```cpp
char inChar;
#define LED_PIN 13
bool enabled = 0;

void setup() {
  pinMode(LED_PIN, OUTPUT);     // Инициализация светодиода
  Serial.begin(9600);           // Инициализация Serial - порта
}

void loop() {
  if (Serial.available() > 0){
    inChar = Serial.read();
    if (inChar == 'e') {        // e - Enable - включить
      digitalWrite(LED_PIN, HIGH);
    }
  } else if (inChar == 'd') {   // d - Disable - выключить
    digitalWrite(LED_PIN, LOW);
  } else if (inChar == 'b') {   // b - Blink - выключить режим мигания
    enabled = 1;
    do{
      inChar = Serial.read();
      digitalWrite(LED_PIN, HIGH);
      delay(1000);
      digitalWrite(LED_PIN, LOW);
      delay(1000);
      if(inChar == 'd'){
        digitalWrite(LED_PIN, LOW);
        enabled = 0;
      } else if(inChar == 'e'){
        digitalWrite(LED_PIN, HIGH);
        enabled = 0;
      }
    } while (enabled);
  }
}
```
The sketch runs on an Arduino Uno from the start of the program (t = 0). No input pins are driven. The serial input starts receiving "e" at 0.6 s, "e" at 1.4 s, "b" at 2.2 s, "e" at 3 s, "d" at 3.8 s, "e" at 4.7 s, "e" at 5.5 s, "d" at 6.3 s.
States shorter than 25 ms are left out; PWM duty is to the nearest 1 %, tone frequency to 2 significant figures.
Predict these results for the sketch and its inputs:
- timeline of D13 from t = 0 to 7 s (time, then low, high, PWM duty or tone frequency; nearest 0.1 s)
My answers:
0 s low; 0.6 s high; 3.2 s low; 4.2 s high; 5.2 s low; 6.2 s high; 6.3 s low
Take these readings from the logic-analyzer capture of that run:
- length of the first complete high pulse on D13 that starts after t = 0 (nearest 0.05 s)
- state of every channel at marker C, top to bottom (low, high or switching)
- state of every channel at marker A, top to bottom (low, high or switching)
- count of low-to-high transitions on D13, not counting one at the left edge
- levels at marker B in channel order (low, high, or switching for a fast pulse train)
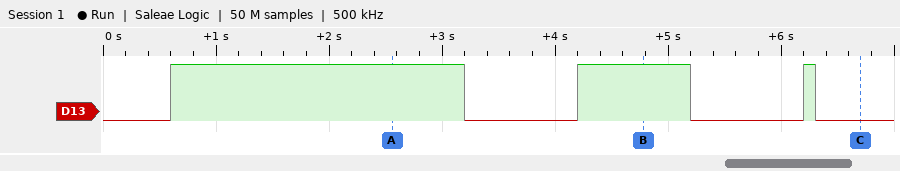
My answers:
2.60 s
D13 low
D13 high
3
D13 high
